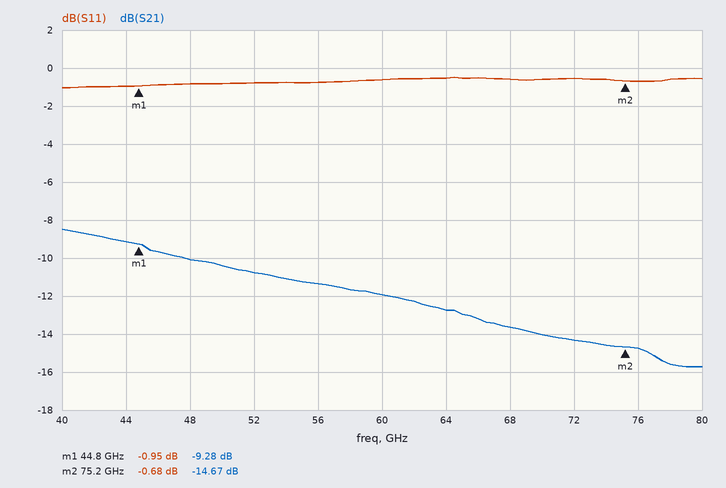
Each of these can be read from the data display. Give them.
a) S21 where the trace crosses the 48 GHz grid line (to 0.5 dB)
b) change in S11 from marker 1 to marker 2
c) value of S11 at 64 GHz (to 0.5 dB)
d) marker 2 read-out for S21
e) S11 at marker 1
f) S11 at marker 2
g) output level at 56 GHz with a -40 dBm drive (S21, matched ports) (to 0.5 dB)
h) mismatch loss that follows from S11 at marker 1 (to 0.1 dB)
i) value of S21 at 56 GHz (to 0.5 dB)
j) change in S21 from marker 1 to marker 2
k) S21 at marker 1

-10.0 dB
0.27 dB
-0.5 dB
-14.67 dB
-0.95 dB
-0.68 dB
-51.5 dBm
7.1 dB
-11.5 dB
-5.39 dB
-9.28 dB
